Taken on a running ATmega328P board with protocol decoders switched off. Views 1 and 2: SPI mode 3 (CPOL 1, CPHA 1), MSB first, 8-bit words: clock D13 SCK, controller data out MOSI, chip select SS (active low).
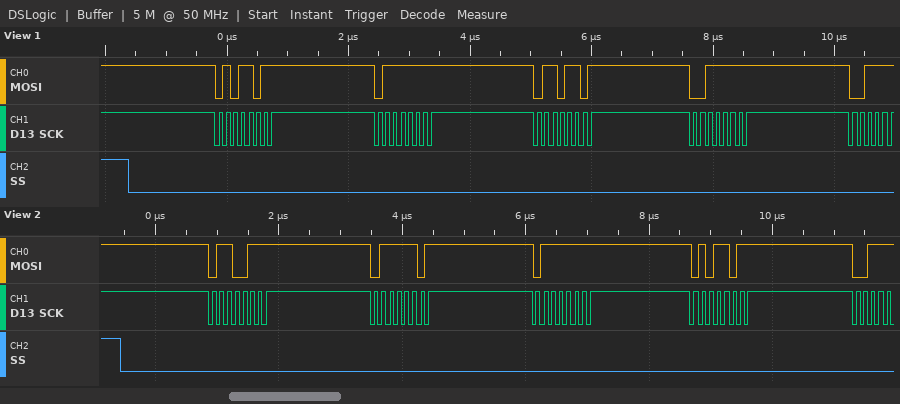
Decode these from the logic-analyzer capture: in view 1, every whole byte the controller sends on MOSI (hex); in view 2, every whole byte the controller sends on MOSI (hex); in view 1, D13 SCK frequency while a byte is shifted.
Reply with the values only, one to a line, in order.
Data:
5B 7F 6D 3F
0x67 0x7D 0x7F 0x5B
8 MHz
